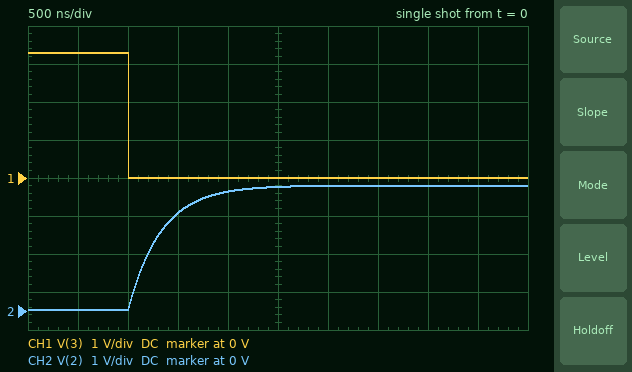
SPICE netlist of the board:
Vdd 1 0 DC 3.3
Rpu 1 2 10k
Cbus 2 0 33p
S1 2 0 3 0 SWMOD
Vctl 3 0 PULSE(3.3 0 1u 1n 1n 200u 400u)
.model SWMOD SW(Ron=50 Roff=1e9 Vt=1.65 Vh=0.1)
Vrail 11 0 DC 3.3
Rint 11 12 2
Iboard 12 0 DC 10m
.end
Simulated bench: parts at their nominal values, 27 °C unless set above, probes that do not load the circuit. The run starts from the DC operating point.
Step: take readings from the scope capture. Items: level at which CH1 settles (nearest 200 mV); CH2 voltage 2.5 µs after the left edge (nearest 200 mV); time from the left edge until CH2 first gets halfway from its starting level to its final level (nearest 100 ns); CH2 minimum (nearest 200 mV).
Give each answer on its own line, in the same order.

0 V
3.2 V
1.2 µs
0 V
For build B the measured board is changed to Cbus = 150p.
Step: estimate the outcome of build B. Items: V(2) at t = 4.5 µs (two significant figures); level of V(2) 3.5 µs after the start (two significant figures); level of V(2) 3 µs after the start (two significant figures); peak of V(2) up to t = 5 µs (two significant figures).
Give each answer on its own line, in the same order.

3.0 V
2.7 V
2.4 V
3.1 V
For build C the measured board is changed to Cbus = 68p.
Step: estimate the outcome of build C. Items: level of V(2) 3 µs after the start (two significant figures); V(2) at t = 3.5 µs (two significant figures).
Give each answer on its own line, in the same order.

3.1 V
3.2 V
